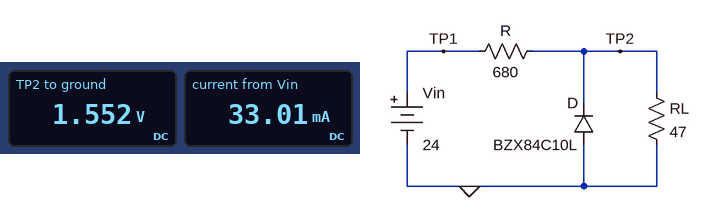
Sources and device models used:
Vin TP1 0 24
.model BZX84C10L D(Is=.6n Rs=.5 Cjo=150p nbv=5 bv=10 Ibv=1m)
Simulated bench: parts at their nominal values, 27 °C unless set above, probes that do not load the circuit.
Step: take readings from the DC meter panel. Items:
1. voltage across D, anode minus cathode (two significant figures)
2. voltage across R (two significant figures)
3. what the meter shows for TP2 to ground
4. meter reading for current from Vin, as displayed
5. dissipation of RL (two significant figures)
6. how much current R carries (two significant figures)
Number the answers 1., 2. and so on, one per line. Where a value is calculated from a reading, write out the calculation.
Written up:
1. 0 V - 1.552 V = -1.6 V
2. 24 V - 1.552 V = 22 V
3. 1.552 V
4. 33.01 mA
5. (1.552 V)^2 / 47 Ω = 51 mW
6. (24 V - 1.552 V) / 680 Ω = 33 mA
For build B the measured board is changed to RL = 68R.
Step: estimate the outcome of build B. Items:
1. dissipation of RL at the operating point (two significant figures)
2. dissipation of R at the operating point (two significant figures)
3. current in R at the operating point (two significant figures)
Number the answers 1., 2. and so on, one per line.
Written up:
1. 70 mW
2. 700 mW
3. 32 mA
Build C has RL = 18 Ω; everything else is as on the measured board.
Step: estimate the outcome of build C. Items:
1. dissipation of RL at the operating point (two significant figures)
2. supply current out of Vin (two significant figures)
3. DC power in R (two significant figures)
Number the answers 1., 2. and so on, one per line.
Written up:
1. 21 mW
2. 34 mA
3. 800 mW
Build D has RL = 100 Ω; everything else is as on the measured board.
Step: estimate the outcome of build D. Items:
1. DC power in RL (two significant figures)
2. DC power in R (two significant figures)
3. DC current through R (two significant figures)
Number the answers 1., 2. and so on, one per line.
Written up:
1. 95 mW
2. 640 mW
3. 31 mA
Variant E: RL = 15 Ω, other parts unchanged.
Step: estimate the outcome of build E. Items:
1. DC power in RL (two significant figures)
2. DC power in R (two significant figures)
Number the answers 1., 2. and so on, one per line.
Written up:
1. 18 mW
2. 810 mW
